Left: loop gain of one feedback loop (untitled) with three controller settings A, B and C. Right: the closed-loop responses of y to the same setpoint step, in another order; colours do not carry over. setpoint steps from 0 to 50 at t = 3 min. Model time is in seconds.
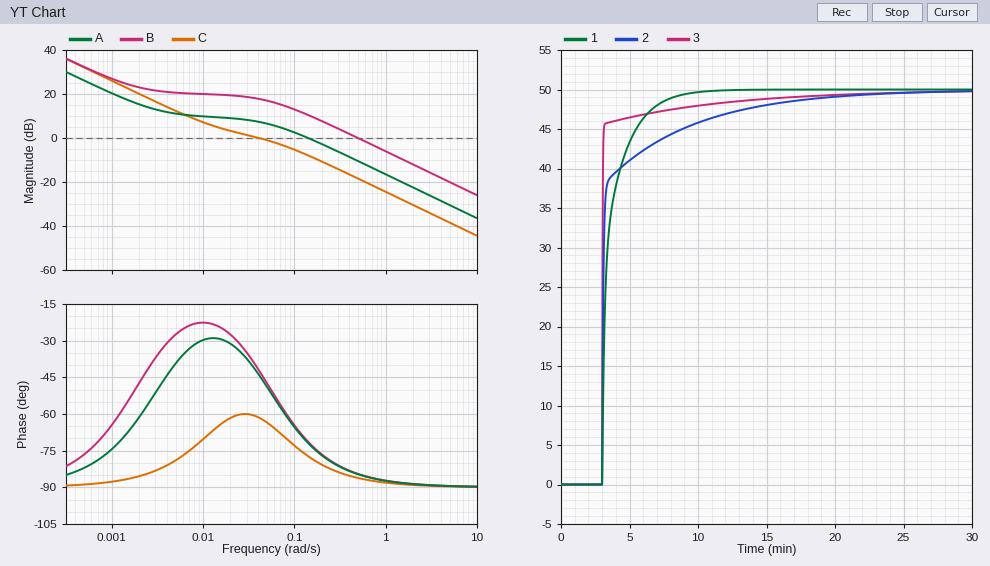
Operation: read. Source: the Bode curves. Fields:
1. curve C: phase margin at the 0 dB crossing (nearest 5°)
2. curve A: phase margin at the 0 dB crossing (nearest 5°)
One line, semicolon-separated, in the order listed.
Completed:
120°; 110°
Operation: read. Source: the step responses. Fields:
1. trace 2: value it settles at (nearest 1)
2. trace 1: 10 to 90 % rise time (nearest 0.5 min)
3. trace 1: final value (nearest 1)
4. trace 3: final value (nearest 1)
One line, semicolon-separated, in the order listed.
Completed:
50; 2.5 min; 50; 50
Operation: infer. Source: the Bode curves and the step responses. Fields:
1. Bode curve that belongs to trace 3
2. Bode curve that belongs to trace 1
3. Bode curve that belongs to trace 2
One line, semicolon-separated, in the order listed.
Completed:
B; C; A
